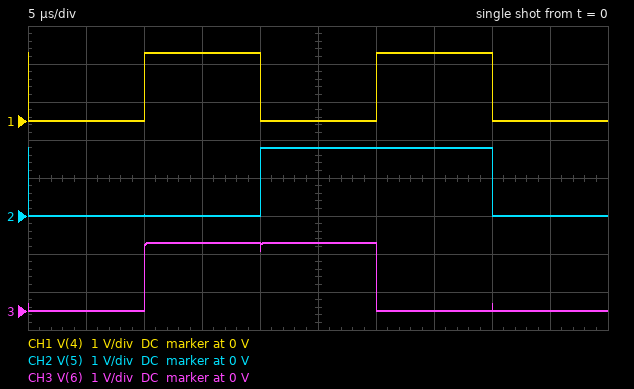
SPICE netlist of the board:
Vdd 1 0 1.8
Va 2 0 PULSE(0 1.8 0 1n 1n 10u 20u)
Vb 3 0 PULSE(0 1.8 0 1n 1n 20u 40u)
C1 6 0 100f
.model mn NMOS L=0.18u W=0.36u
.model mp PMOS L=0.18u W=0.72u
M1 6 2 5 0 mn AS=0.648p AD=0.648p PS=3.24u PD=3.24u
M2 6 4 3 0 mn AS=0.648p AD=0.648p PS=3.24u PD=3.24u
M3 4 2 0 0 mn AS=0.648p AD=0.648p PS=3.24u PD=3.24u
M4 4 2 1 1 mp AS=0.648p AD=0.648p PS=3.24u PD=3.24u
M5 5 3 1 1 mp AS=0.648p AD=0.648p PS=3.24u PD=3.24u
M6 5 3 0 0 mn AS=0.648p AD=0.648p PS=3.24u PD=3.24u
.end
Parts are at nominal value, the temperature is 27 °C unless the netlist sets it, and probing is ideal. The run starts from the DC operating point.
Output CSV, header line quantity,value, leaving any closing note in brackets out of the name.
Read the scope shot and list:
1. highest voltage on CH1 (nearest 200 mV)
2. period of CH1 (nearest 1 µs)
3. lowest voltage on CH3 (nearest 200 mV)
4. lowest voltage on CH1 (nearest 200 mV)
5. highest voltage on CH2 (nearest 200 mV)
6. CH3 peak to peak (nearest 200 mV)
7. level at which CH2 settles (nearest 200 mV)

quantity,value
highest voltage on CH1,1.8 V
period of CH1,20 µs
lowest voltage on CH3,0 V
lowest voltage on CH1,0 V
highest voltage on CH2,1.8 V
CH3 peak to peak,1.8 V
level at which CH2 settles,0 V
